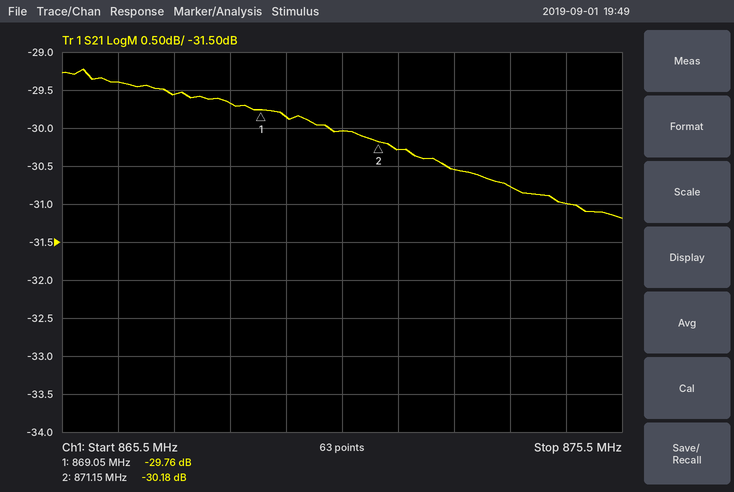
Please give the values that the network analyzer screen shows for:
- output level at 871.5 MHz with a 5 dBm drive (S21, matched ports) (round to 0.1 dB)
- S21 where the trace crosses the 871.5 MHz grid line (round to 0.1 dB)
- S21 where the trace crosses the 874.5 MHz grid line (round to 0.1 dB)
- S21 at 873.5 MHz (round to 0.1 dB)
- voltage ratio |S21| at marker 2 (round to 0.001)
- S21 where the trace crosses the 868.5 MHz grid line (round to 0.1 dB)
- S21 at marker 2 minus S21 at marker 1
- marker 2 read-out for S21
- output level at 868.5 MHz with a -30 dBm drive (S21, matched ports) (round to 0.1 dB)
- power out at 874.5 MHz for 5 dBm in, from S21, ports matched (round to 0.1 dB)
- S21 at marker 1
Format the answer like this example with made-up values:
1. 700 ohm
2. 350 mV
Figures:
1. -25.3 dBm
2. -30.3 dB
3. -31.0 dB
4. -30.8 dB
5. 0.031
6. -29.7 dB
7. -0.42 dB
8. -30.18 dB
9. -59.7 dBm
10. -26.0 dBm
11. -29.76 dB
